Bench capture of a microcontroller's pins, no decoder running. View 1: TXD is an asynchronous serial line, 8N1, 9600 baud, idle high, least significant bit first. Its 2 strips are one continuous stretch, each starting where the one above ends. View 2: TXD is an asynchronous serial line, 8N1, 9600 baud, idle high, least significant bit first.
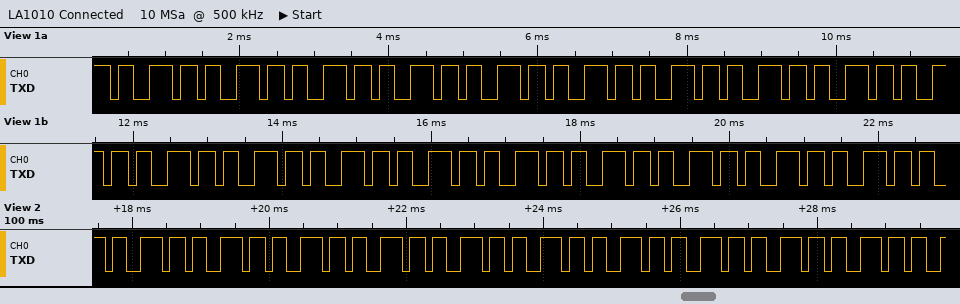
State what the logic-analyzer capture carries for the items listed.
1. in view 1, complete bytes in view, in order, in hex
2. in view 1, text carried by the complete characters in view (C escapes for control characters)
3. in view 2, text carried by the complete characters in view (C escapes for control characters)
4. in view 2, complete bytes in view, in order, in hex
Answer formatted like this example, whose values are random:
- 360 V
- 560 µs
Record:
- 0x73 0x73 0x73 0x73 0x73 0x73 0x73 0x73 0x73 0x73 0x73 0x73 0x73 0x73 0x73 0x73 0x73 0x73 0x73
- "sssssssssssssssssss"
- "ssssssssss"
- 73 73 73 73 73 73 73 73 73 73
